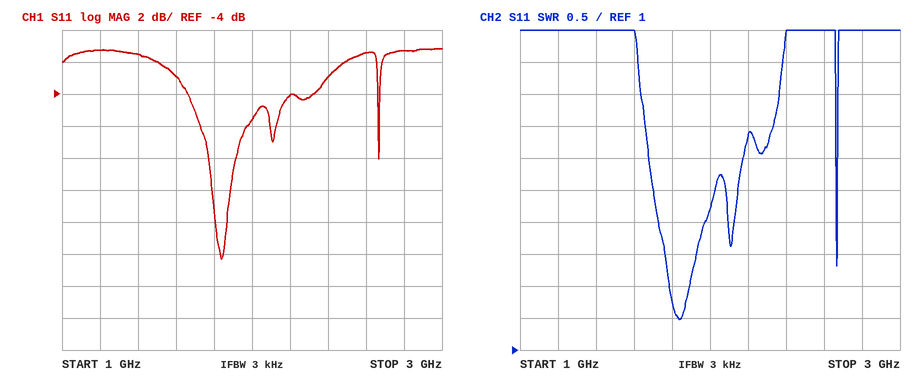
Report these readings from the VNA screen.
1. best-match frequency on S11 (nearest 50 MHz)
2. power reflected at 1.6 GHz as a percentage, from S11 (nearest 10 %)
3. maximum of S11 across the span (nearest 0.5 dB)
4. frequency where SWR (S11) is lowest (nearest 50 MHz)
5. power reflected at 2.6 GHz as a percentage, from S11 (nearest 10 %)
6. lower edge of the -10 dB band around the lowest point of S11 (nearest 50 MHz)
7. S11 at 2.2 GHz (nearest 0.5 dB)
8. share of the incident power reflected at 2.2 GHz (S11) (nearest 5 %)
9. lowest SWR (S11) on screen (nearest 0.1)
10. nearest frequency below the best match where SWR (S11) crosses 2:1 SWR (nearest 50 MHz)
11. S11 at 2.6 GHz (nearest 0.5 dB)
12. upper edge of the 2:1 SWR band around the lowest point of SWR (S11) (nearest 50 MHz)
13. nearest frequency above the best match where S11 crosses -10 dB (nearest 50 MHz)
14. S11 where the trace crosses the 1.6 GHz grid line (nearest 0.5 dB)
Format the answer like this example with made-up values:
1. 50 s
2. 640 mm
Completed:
1. 1.85 GHz
2. 50 %
3. -1.0 dB
4. 1.85 GHz
5. 70 %
6. 1.80 GHz
7. -4.0 dB
8. 40 %
9. 1.5
10. 1.80 GHz
11. -1.5 dB
12. 1.90 GHz
13. 1.90 GHz
14. -3.0 dB
